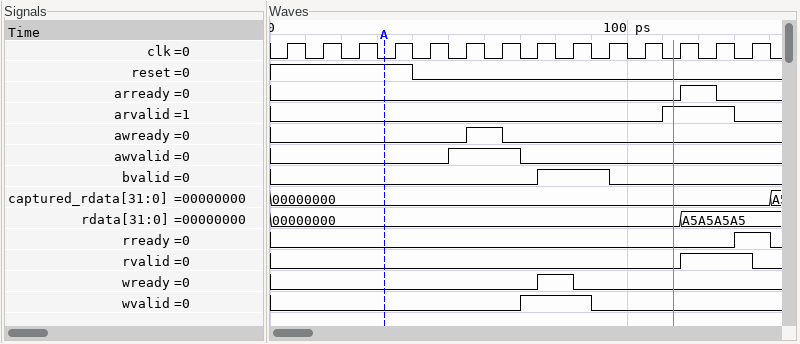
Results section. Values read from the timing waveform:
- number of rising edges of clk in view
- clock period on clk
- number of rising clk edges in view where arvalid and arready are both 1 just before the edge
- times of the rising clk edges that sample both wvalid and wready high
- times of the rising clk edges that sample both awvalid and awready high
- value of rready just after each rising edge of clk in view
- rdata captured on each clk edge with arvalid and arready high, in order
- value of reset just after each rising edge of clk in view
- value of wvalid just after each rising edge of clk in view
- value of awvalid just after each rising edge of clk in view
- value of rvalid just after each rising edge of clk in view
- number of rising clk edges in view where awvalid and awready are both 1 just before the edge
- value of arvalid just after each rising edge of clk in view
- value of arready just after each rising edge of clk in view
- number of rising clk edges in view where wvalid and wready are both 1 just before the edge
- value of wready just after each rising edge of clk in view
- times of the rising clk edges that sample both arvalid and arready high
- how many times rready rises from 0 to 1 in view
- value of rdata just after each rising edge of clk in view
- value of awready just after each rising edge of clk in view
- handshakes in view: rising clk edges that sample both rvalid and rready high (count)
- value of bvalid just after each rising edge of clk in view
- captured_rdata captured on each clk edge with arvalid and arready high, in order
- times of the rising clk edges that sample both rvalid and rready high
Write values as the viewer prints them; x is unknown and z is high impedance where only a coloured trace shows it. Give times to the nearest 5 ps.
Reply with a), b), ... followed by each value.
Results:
a) 14
b) 10 ps
c) 1
d) 85 ps
e) 65 ps
f) 0 0 0 0 0 0 0 0 0 0 0 0 0 1
g) A5A5A5A5
h) 1 1 1 1 0 0 0 0 0 0 0 0 0 0
i) 0 0 0 0 0 0 0 1 1 0 0 0 0 0
j) 0 0 0 0 0 1 1 0 0 0 0 0 0 0
k) 0 0 0 0 0 0 0 0 0 0 0 1 1 0
l) 1
m) 0 0 0 0 0 0 0 0 0 0 0 1 1 0
n) 0 0 0 0 0 0 0 0 0 0 0 1 0 0
o) 1
p) 0 0 0 0 0 0 0 1 0 0 0 0 0 0
q) 125 ps
r) 1
s) 00000000, 00000000, 00000000, 00000000, 00000000, 00000000, 00000000, 00000000, 00000000, 00000000, 00000000, A5A5A5A5, A5A5A5A5, A5A5A5A5
t) 0 0 0 0 0 1 0 0 0 0 0 0 0 0
u) 1
v) 0 0 0 0 0 0 0 1 1 0 0 0 0 0
w) 00000000
x) 135 ps
